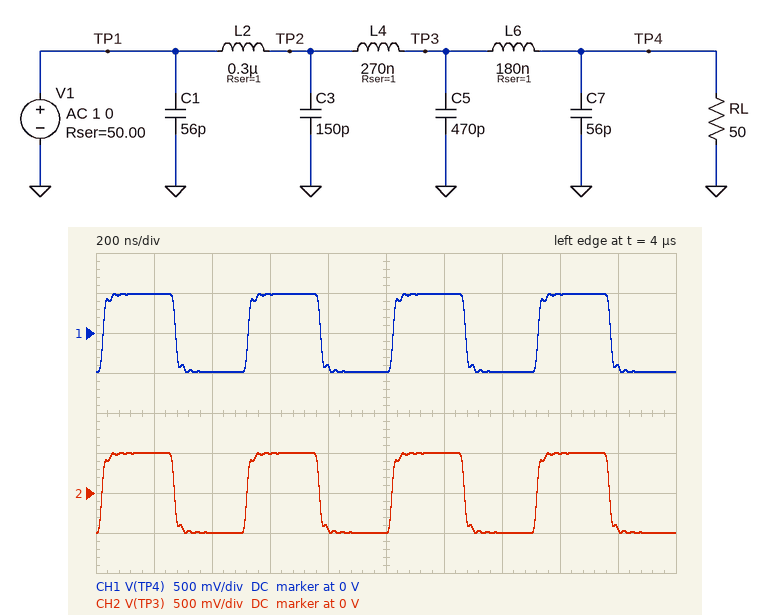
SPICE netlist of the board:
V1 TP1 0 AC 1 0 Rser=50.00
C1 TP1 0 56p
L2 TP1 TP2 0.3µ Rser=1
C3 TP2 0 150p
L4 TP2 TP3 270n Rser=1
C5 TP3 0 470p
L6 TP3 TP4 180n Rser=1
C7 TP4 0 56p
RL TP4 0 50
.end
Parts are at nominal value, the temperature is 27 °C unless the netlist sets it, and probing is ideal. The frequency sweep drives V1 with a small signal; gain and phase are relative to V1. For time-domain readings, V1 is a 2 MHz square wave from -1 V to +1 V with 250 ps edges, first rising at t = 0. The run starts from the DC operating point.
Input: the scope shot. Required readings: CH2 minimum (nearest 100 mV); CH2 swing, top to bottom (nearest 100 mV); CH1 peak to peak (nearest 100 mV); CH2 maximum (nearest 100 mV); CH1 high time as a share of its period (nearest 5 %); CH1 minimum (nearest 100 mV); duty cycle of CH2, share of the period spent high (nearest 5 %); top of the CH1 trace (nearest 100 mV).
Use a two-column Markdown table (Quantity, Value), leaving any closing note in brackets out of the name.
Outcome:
| Quantity | Value |
|---|---|
| CH2 minimum | -500 mV |
| CH2 swing, top to bottom | 1.0 V |
| CH1 peak to peak | 1.0 V |
| CH2 maximum | 500 mV |
| CH1 high time as a share of its period | 50 % |
| CH1 minimum | -500 mV |
| duty cycle of CH2, share of the period spent high | 50 % |
| top of the CH1 trace | 500 mV |
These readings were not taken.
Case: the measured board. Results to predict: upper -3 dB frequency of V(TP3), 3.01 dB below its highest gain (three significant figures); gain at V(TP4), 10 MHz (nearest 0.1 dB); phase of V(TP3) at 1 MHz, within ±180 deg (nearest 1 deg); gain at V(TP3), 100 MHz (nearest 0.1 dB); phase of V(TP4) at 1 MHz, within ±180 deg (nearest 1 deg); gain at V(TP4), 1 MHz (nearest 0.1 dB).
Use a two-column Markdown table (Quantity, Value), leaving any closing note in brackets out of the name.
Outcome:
| Quantity | Value |
|---|---|
| upper -3 dB frequency of V(TP3), 3.01 dB below its highest gain | 15.1 MHz |
| gain at V(TP4), 10 MHz | -7.9 dB |
| phase of V(TP3) at 1 MHz, within ±180 deg | -8 deg |
| gain at V(TP3), 100 MHz | -62.4 dB |
| phase of V(TP4) at 1 MHz, within ±180 deg | -9 deg |
| gain at V(TP4), 1 MHz | -6.3 dB |
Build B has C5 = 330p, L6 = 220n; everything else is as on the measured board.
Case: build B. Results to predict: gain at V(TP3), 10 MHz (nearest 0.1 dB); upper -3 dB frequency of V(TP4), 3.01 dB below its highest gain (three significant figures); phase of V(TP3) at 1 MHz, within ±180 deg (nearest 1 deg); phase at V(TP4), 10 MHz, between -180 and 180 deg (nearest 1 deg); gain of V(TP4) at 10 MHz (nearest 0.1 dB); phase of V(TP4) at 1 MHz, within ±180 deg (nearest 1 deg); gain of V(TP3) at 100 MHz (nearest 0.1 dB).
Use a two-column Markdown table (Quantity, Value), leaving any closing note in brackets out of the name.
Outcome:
| Quantity | Value |
|---|---|
| gain at V(TP3), 10 MHz | -6.9 dB |
| upper -3 dB frequency of V(TP4), 3.01 dB below its highest gain | 35.6 MHz |
| phase of V(TP3) at 1 MHz, within ±180 deg | -7 deg |
| phase at V(TP4), 10 MHz, between -180 and 180 deg | -81 deg |
| gain of V(TP4) at 10 MHz | -7.0 dB |
| phase of V(TP4) at 1 MHz, within ±180 deg | -8 deg |
| gain of V(TP3) at 100 MHz | -59.2 dB |
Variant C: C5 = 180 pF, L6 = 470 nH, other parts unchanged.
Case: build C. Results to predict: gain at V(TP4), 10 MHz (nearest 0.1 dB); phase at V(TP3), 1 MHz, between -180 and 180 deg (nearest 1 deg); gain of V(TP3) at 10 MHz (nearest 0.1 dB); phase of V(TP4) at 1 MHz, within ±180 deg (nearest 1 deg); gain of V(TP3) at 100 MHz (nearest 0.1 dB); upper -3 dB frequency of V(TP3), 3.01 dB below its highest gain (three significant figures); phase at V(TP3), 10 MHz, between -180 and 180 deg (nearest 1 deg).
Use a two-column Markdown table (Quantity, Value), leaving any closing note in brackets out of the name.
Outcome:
| Quantity | Value |
|---|---|
| gain at V(TP4), 10 MHz | -6.3 dB |
| phase at V(TP3), 1 MHz, between -180 and 180 deg | -4 deg |
| gain of V(TP3) at 10 MHz | -5.6 dB |
| phase of V(TP4) at 1 MHz, within ±180 deg | -8 deg |
| gain of V(TP3) at 100 MHz | -53.8 dB |
| upper -3 dB frequency of V(TP3), 3.01 dB below its highest gain | 43.0 MHz |
| phase at V(TP3), 10 MHz, between -180 and 180 deg | -45 deg |
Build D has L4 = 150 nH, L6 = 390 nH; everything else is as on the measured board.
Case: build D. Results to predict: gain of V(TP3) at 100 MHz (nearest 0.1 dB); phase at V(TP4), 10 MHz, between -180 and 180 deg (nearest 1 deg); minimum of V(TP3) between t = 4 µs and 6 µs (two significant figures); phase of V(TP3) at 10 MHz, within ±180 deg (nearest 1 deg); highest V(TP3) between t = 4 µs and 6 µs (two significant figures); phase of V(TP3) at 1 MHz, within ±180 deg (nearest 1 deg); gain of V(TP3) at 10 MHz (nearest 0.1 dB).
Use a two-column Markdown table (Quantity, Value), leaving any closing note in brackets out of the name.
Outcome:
| Quantity | Value |
|---|---|
| gain of V(TP3) at 100 MHz | -56.8 dB |
| phase at V(TP4), 10 MHz, between -180 and 180 deg | -94 deg |
| minimum of V(TP3) between t = 4 µs and 6 µs | -520 mV |
| phase of V(TP3) at 10 MHz, within ±180 deg | -66 deg |
| highest V(TP3) between t = 4 µs and 6 µs | 520 mV |
| phase of V(TP3) at 1 MHz, within ±180 deg | -7 deg |
| gain of V(TP3) at 10 MHz | -7.4 dB |
